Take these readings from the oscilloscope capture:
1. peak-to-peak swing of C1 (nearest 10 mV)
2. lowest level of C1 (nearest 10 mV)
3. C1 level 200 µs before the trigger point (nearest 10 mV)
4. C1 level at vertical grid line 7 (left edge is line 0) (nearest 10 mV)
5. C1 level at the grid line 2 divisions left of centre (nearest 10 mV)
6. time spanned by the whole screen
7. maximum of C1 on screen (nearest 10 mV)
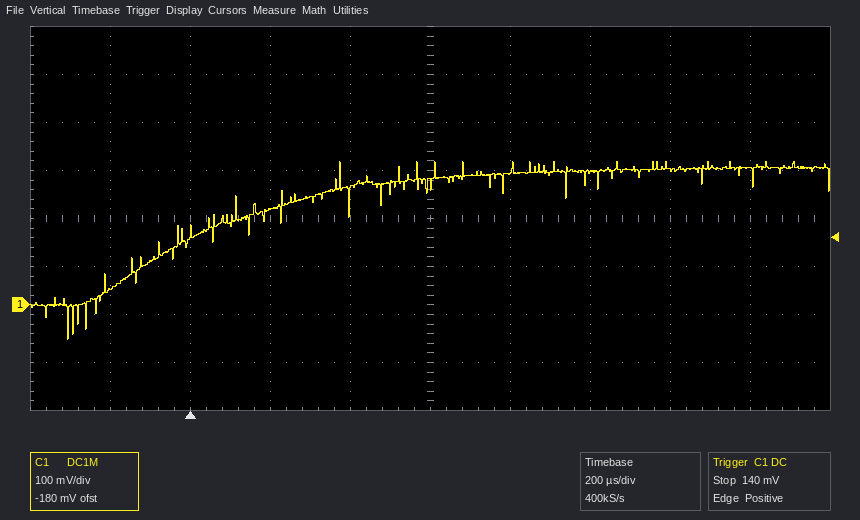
370 mV
-70 mV
30 mV
280 mV
200 mV
2 ms
300 mV
